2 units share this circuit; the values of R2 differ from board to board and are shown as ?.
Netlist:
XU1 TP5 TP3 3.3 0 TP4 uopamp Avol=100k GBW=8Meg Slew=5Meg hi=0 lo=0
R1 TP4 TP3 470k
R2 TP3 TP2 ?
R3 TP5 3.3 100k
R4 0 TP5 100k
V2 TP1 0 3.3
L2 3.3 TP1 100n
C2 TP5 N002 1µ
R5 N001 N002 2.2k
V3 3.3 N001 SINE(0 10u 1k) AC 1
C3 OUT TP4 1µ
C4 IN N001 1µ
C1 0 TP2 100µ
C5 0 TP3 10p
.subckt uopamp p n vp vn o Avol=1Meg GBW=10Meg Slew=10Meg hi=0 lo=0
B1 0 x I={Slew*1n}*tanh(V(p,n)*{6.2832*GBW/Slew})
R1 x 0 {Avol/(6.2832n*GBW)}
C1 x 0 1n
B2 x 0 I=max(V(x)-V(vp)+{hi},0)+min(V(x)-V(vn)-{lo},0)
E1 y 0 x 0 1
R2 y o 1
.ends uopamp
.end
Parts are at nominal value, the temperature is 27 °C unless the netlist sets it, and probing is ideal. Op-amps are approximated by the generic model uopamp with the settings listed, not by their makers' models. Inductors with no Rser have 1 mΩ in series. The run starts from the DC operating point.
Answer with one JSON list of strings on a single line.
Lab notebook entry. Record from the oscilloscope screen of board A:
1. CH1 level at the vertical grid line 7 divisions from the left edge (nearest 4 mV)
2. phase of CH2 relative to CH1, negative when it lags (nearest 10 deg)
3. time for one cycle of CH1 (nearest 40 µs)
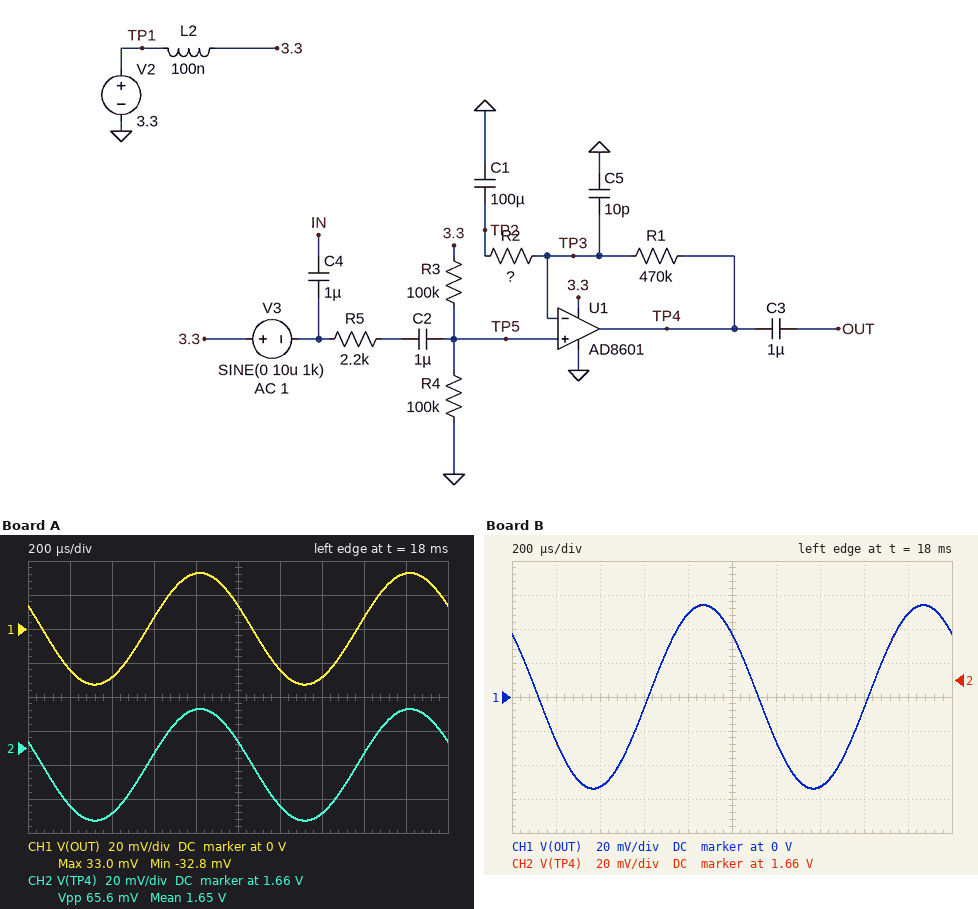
["-28 mV", "0 deg", "1.00 ms"]
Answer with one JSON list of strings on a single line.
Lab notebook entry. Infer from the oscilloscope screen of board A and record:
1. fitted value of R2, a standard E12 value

["120 Ω"]
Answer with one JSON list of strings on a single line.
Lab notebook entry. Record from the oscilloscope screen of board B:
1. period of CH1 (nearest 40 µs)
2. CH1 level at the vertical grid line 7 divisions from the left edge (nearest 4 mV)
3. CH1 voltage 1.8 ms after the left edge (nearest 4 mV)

["1.00 ms", "-52 mV", "48 mV"]
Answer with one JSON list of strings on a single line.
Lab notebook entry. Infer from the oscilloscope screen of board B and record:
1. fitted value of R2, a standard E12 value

["56 Ω"]
